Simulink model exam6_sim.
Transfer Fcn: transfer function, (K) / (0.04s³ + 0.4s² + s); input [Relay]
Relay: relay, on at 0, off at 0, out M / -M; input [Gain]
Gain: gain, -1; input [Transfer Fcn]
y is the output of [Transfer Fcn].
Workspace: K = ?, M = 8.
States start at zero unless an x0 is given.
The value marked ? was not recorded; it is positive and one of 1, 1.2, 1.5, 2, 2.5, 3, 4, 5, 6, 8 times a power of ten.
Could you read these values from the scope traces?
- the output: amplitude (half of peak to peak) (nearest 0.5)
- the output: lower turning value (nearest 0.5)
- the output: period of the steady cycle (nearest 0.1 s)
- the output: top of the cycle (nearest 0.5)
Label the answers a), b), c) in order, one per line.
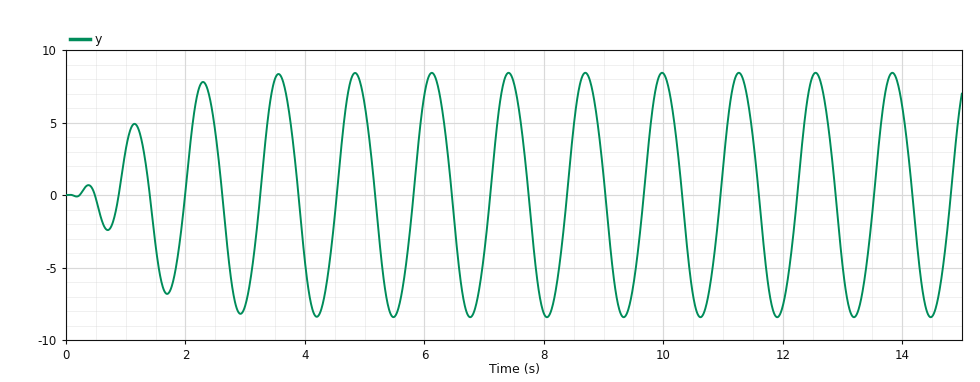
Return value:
a) 8.5
b) -8.5
c) 1.3 s
d) 8.5
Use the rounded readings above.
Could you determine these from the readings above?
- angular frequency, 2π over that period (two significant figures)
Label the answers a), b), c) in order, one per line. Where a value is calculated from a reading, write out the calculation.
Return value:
a) 2π / 1.3 = 4.8 rad/s
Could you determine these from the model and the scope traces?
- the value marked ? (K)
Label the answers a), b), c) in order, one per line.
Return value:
a) 8
